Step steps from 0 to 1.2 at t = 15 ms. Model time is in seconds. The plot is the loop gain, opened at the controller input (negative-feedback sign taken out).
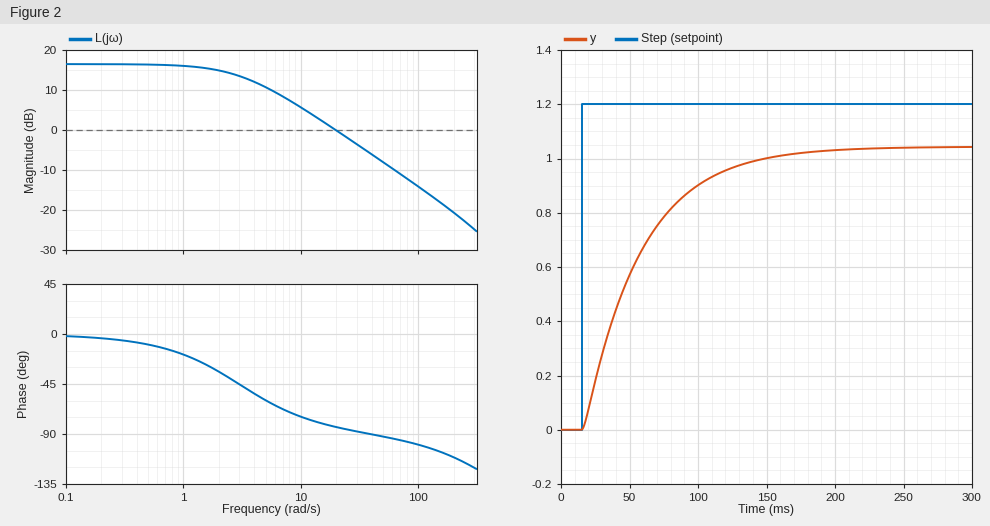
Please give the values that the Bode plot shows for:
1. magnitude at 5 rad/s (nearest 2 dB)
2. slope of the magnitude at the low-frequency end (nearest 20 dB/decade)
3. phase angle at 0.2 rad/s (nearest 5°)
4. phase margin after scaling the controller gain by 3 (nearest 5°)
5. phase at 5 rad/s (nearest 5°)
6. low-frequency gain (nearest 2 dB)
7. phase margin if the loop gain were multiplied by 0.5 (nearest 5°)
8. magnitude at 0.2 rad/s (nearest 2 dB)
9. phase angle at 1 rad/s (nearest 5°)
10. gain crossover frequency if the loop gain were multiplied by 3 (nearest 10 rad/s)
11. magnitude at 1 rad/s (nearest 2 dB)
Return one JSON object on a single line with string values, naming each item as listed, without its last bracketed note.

{"magnitude at 5 rad/s": "10 dB", "slope of the magnitude at the low-frequency end": "0 dB/decade", "phase angle at 0.2 rad/s": "-5°", "phase margin after scaling the controller gain by 3": "85°", "phase at 5 rad/s": "-60°", "low-frequency gain": "16 dB", "phase margin if the loop gain were multiplied by 0.5": "105°", "magnitude at 0.2 rad/s": "16 dB", "phase angle at 1 rad/s": "-20°", "gain crossover frequency if the loop gain were multiplied by 3": "60 rad/s", "magnitude at 1 rad/s": "16 dB"}
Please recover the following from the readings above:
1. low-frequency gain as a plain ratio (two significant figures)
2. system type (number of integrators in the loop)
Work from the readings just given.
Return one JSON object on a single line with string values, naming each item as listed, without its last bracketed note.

{"low-frequency gain as a plain ratio": "6.3", "system type": "0"}
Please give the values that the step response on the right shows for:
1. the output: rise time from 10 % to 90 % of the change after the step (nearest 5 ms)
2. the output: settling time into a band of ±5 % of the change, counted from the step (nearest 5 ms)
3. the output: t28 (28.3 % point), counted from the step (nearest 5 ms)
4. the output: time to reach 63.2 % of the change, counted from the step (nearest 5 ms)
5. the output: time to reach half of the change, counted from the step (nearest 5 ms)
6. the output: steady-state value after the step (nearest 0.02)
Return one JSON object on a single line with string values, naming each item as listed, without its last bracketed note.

{"the output: rise time from 10 % to 90 % of the change after the step": "90 ms", "the output: settling time into a band of ±5 % of the change, counted from the step": "125 ms", "the output: t28 (28.3 % point), counted from the step": "15 ms", "the output: time to reach 63.2 % of the change, counted from the step": "45 ms", "the output: time to reach half of the change, counted from the step": "30 ms", "the output: steady-state value after the step": "1.04"}
